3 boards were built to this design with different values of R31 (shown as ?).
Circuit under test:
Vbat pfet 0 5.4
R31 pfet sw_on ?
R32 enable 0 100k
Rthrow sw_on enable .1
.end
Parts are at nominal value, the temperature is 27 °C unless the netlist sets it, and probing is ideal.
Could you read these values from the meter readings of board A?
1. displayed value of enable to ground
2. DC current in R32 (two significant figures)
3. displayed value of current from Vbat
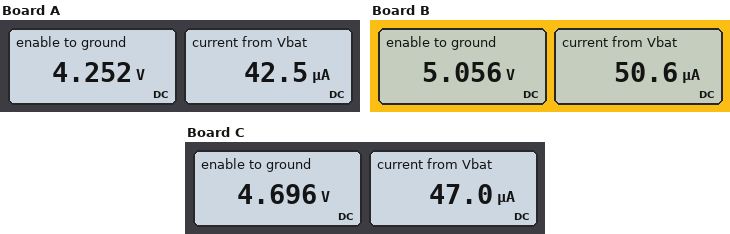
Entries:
4.252 V
43 µA
42.5 µA
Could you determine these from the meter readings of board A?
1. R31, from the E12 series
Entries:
27 kΩ
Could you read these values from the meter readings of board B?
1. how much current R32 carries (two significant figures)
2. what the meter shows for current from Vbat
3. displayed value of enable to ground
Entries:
51 µA
50.6 µA
5.056 V
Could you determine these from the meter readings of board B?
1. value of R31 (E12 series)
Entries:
6.8 kΩ
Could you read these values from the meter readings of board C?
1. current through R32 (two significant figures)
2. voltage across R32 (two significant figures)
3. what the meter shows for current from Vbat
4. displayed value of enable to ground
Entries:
47 µA
4.7 V
47.0 µA
4.696 V
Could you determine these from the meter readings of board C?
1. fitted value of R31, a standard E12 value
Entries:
15 kΩ
